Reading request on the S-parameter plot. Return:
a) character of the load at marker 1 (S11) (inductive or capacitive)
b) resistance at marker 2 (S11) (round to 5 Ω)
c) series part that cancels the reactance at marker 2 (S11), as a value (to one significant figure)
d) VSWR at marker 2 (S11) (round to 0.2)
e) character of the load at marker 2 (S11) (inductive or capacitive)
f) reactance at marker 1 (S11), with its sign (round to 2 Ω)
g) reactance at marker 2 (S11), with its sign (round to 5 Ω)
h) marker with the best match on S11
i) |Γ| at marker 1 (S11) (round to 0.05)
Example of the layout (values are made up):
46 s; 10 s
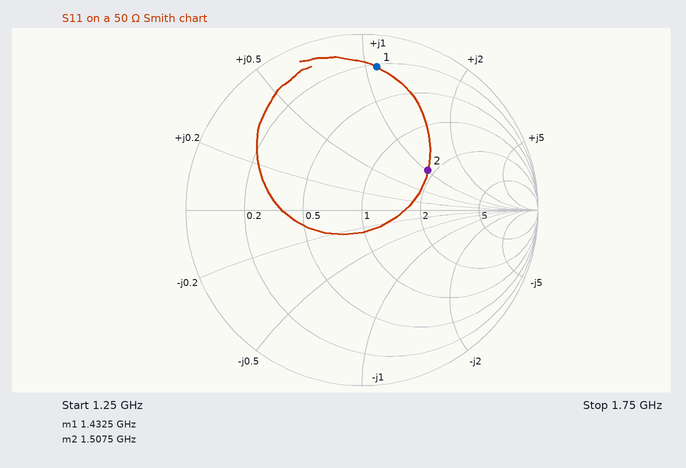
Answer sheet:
inductive; 90 Ω; 2 pF; 2.6; inductive; +54 Ω; +50 Ω; marker 2; 0.80
